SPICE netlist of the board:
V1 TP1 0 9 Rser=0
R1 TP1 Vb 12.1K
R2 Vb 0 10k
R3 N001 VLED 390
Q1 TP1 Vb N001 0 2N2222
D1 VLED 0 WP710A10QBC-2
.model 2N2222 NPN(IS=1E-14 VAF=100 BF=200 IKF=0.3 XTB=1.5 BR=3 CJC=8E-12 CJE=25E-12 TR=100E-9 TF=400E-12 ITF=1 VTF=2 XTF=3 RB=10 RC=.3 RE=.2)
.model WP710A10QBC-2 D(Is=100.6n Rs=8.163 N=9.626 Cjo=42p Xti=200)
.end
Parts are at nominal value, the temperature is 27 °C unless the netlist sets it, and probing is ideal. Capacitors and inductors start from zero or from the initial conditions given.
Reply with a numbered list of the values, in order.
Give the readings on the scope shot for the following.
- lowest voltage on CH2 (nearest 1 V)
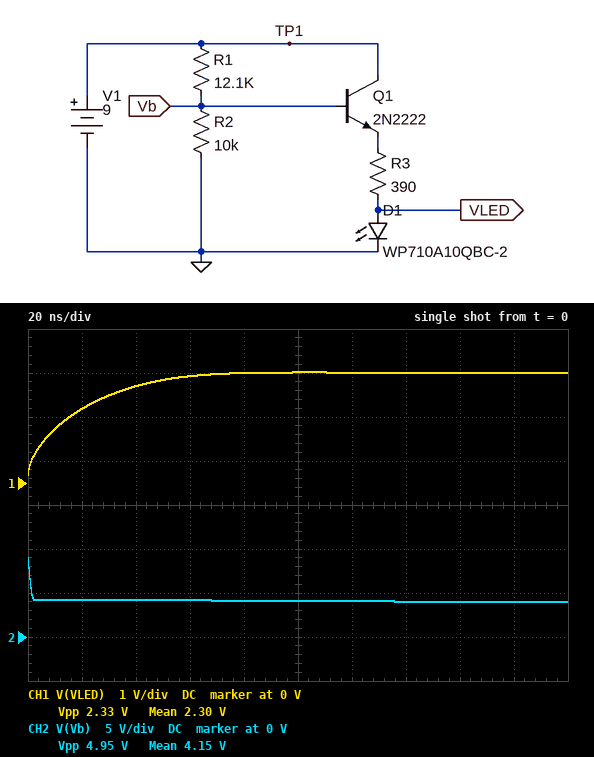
1. 4 V
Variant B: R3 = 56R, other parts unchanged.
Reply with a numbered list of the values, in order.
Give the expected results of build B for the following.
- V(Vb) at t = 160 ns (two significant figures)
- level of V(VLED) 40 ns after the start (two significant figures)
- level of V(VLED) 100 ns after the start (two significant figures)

1. 3.9 V
2. 2.9 V
3. 2.8 V
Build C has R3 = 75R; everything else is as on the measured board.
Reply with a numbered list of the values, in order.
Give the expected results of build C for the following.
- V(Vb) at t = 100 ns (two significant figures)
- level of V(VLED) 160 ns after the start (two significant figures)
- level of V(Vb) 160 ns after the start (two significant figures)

1. 4.0 V
2. 2.8 V
3. 3.9 V
